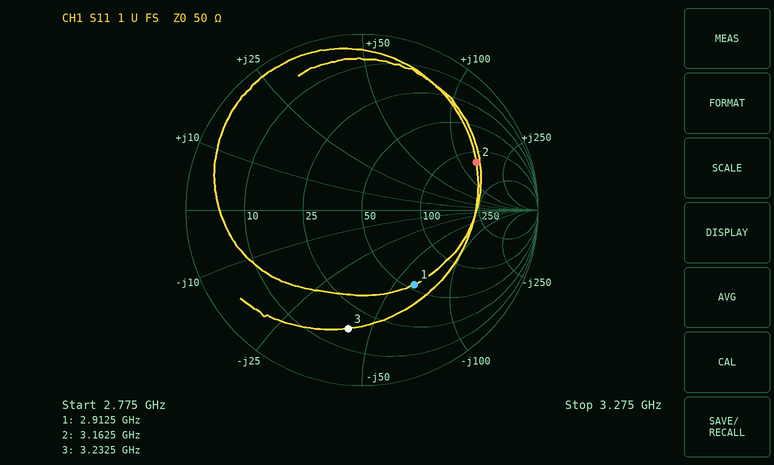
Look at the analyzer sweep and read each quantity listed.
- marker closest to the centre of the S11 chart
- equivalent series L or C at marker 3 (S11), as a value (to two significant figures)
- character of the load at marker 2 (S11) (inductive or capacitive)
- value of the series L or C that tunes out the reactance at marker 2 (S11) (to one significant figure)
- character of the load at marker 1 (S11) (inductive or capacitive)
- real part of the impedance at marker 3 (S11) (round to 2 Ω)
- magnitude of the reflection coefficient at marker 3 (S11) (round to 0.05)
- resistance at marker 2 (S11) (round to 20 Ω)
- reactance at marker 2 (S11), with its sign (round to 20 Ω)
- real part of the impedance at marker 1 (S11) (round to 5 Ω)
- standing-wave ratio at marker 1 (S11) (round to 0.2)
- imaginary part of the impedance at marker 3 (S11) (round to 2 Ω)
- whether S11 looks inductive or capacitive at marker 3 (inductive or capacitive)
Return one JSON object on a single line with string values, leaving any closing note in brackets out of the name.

{"marker closest to the centre of the S11 chart": "marker 1", "equivalent series L or C at marker 3 (S11), as a value": "1.2 pF", "character of the load at marker 2 (S11)": "inductive", "value of the series L or C that tunes out the reactance at marker 2 (S11)": "400 fF", "character of the load at marker 1 (S11)": "capacitive", "real part of the impedance at marker 3 (S11)": "16 Ω", "magnitude of the reflection coefficient at marker 3 (S11)": "0.70", "resistance at marker 2 (S11)": "120 Ω", "reactance at marker 2 (S11), with its sign": "+140 Ω", "real part of the impedance at marker 1 (S11)": "55 Ω", "standing-wave ratio at marker 1 (S11)": "3.2", "imaginary part of the impedance at marker 3 (S11)": "-42 Ω", "whether S11 looks inductive or capacitive at marker 3": "capacitive"}
